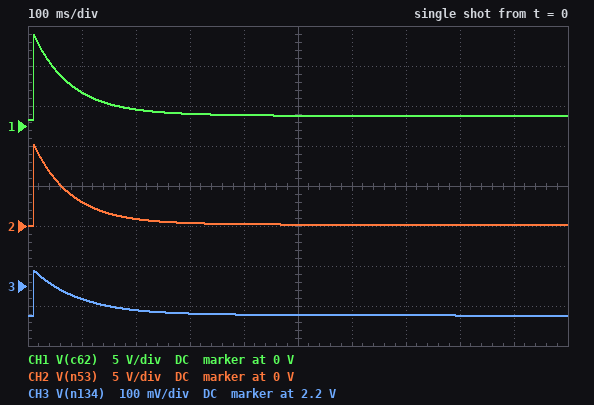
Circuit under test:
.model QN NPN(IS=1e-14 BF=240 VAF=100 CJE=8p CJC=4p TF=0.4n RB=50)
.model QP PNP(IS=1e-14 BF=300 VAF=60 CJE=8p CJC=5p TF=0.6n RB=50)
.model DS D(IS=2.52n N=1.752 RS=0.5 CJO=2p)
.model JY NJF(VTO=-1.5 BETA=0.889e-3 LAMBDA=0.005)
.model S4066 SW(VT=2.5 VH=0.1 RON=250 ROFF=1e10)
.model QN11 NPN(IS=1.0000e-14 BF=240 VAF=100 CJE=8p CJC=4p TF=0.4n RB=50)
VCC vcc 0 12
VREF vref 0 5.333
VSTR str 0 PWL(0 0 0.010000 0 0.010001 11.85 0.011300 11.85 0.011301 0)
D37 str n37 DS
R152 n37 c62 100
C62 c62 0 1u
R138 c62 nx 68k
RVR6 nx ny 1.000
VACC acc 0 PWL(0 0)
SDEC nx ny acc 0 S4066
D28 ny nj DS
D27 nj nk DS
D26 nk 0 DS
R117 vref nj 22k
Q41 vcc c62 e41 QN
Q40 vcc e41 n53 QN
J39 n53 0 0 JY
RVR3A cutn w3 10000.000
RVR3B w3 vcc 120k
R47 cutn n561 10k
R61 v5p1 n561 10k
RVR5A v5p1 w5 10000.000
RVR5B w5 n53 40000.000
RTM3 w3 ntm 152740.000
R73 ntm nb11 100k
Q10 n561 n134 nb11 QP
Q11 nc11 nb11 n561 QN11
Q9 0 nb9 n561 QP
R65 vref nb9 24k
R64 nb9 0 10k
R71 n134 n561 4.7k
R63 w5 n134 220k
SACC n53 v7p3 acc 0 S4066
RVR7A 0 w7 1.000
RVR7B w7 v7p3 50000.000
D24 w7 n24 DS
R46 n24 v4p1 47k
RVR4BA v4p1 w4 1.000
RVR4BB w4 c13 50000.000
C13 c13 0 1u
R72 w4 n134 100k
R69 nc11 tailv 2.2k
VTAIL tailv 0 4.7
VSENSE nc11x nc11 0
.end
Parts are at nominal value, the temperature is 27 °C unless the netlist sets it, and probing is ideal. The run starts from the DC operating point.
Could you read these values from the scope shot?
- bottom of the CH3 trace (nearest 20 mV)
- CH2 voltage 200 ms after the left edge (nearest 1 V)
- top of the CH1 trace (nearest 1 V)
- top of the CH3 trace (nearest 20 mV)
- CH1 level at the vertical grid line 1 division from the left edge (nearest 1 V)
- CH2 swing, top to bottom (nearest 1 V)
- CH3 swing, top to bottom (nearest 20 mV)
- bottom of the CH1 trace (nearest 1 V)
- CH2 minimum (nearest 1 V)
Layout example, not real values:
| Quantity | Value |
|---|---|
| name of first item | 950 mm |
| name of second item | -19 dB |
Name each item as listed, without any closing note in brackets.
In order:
| Quantity | Value |
|---|---|
| bottom of the CH3 trace | 2.12 V |
| CH2 voltage 200 ms after the left edge | 1 V |
| top of the CH1 trace | 11 V |
| top of the CH3 trace | 2.24 V |
| CH1 level at the vertical grid line 1 division from the left edge | 4 V |
| CH2 swing, top to bottom | 10 V |
| CH3 swing, top to bottom | 120 mV |
| bottom of the CH1 trace | 1 V |
| CH2 minimum | 0 V |
